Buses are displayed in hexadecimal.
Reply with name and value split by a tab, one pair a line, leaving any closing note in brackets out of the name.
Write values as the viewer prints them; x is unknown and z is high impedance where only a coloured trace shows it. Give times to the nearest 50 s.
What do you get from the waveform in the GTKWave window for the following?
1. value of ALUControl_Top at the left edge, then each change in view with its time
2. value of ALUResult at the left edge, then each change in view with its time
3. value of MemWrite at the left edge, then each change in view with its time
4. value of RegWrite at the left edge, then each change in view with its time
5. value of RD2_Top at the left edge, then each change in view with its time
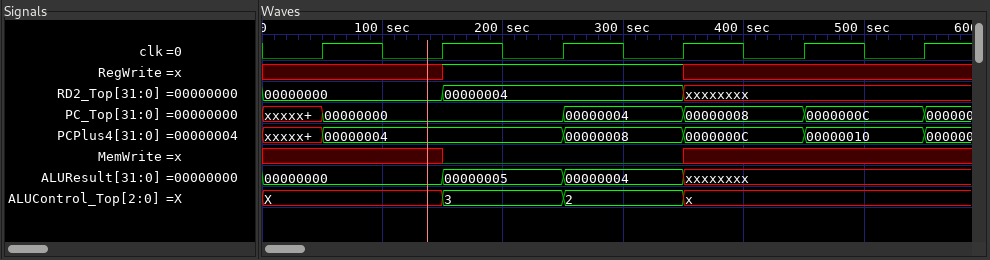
value of ALUControl_Top at the left edge, then each change in view with its time	X, 3 at 150 s, 2 at 250 s, x at 350 s
value of ALUResult at the left edge, then each change in view with its time	00000000, 00000005 at 150 s, 00000004 at 250 s, xxxxxxxx at 350 s
value of MemWrite at the left edge, then each change in view with its time	x, 0 at 150 s, x at 350 s
value of RegWrite at the left edge, then each change in view with its time	x, 1 at 150 s, x at 350 s
value of RD2_Top at the left edge, then each change in view with its time	00000000, 00000004 at 150 s, xxxxxxxx at 350 s
